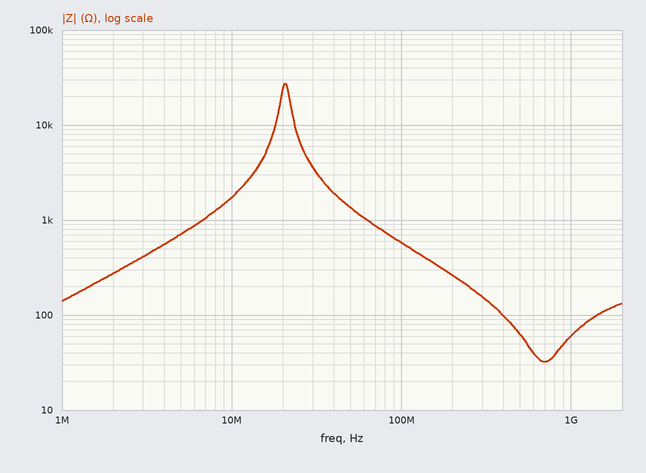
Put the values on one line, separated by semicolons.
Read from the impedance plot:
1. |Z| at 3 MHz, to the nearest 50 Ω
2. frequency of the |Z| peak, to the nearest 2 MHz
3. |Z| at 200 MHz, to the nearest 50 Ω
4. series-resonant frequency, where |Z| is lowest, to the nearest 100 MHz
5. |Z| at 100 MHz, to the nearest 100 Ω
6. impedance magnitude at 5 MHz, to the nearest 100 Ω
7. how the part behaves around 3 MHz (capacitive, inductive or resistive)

400 Ω; 20 MHz; 250 Ω; 700 MHz; 600 Ω; 700 Ω; inductive
